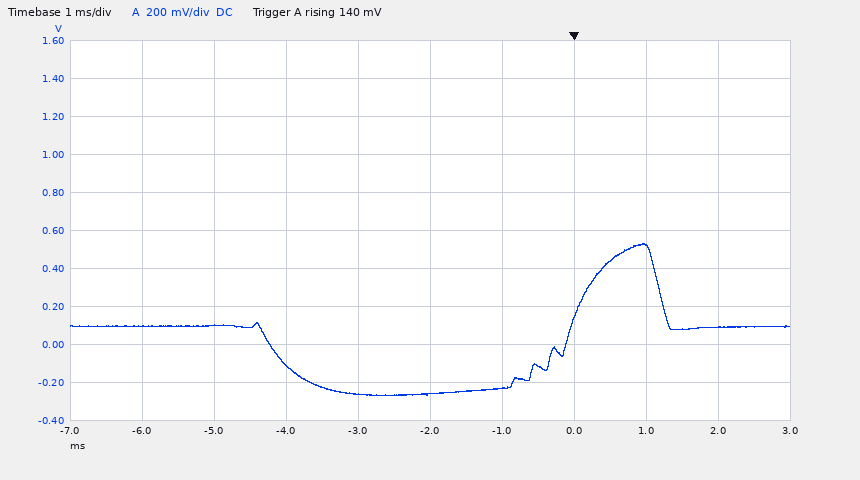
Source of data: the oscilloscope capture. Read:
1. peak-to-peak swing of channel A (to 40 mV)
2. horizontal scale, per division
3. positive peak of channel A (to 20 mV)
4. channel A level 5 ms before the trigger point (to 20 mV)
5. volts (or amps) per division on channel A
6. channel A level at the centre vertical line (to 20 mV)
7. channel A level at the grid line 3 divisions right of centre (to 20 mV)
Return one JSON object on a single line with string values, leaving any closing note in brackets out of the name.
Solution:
{"peak-to-peak swing of channel A": "800 mV", "horizontal scale, per division": "1 ms", "positive peak of channel A": "540 mV", "channel A level 5 ms before the trigger point": "100 mV", "volts (or amps) per division on channel A": "200 mV", "channel A level at the centre vertical line": "-260 mV", "channel A level at the grid line 3 divisions right of centre": "520 mV"}
